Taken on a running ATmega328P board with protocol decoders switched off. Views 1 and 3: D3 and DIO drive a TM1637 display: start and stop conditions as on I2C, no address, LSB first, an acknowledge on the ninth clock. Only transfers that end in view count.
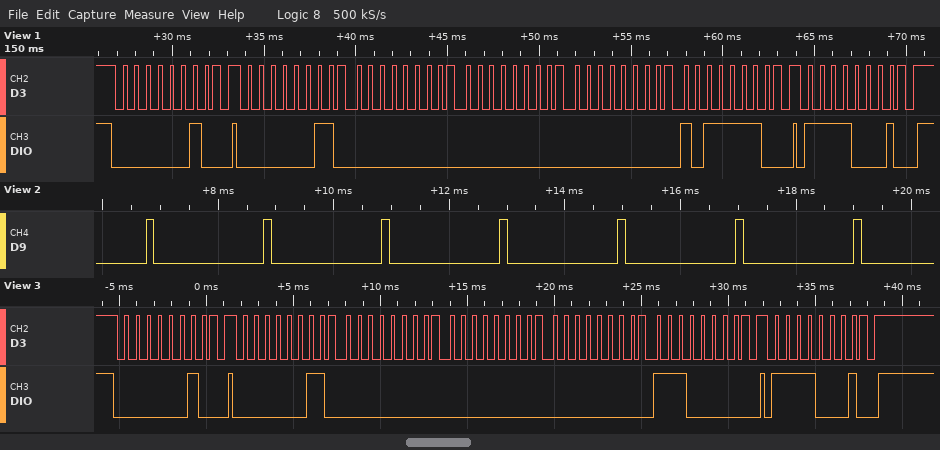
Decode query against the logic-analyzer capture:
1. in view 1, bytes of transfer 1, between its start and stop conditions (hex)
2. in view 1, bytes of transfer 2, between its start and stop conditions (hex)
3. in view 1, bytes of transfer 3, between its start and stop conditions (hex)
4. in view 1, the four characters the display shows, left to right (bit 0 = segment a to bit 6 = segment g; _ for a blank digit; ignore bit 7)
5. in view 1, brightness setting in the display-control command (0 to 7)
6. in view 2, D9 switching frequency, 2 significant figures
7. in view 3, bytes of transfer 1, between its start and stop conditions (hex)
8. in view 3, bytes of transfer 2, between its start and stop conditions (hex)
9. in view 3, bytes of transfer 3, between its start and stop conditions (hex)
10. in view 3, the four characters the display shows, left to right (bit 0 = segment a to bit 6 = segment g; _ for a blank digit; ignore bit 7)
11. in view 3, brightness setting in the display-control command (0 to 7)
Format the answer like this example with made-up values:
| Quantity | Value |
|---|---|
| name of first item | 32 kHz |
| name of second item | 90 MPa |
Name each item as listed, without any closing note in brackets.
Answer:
| Quantity | Value |
|---|---|
| in view 1, bytes of transfer 1, between its start and stop conditions | 40 |
| in view 1, bytes of transfer 2, between its start and stop conditions | C0 00 00 00 7D |
| in view 1, bytes of transfer 3, between its start and stop conditions | 8F |
| in view 1, the four characters the display shows, left to right | ___6 |
| in view 1, brightness setting in the display-control command | 7 |
| in view 2, D9 switching frequency, 2 significant figures | 490 Hz |
| in view 3, bytes of transfer 1, between its start and stop conditions | 40 |
| in view 3, bytes of transfer 2, between its start and stop conditions | C0 00 00 00 07 |
| in view 3, bytes of transfer 3, between its start and stop conditions | 8F |
| in view 3, the four characters the display shows, left to right | ___7 |
| in view 3, brightness setting in the display-control command | 7 |
